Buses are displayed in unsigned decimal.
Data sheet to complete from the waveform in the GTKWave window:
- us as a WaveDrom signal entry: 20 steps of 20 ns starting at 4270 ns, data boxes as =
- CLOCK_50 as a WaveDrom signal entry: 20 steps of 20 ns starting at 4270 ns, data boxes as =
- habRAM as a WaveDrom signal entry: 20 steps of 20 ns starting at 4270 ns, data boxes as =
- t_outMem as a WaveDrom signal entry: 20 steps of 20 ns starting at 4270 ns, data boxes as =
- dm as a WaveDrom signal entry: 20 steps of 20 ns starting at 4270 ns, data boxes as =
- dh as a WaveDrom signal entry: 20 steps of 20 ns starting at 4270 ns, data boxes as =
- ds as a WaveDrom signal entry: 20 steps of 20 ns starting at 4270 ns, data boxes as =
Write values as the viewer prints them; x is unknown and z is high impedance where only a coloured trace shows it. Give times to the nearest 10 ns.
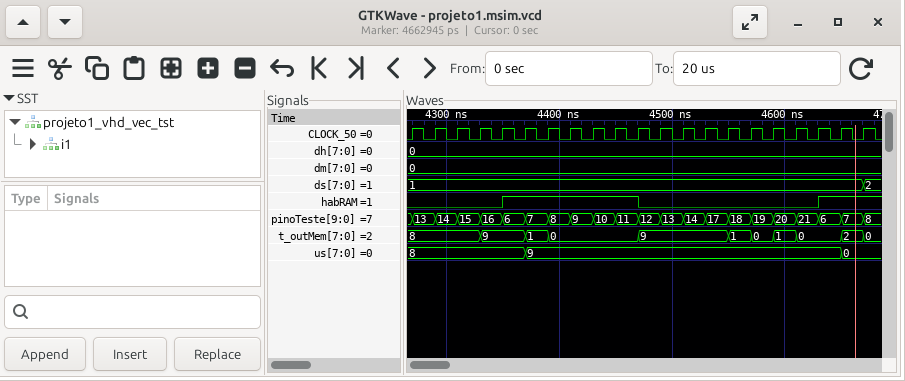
{name: 'us', wave: '=....=.............=', data: '8 9 0'}
{name: 'CLOCK_50', wave: 'p...................'}
{name: 'habRAM', wave: '0...1.....0.......1.'}
{name: 't_outMem', wave: '=..=.==...=...====.=', data: '8 9 1 0 9 1 0 1 0 2'}
{name: 'dm', wave: '=...................', data: '0'}
{name: 'dh', wave: '=...................', data: '0'}
{name: 'ds', wave: '=...................', data: '1'}
